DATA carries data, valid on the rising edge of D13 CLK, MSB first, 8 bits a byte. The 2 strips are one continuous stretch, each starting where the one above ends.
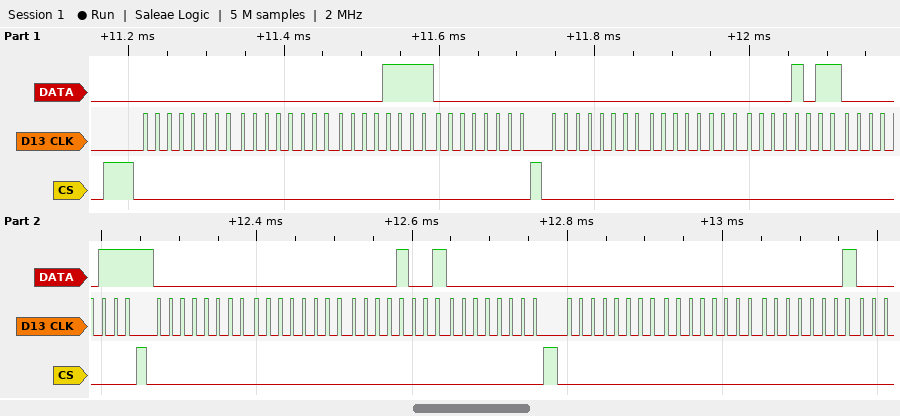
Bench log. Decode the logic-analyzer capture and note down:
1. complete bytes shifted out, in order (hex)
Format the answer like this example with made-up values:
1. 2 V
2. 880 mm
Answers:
1. 00 00 0F 00 00 00 0B 07 00 00 09 00 00 00 01
